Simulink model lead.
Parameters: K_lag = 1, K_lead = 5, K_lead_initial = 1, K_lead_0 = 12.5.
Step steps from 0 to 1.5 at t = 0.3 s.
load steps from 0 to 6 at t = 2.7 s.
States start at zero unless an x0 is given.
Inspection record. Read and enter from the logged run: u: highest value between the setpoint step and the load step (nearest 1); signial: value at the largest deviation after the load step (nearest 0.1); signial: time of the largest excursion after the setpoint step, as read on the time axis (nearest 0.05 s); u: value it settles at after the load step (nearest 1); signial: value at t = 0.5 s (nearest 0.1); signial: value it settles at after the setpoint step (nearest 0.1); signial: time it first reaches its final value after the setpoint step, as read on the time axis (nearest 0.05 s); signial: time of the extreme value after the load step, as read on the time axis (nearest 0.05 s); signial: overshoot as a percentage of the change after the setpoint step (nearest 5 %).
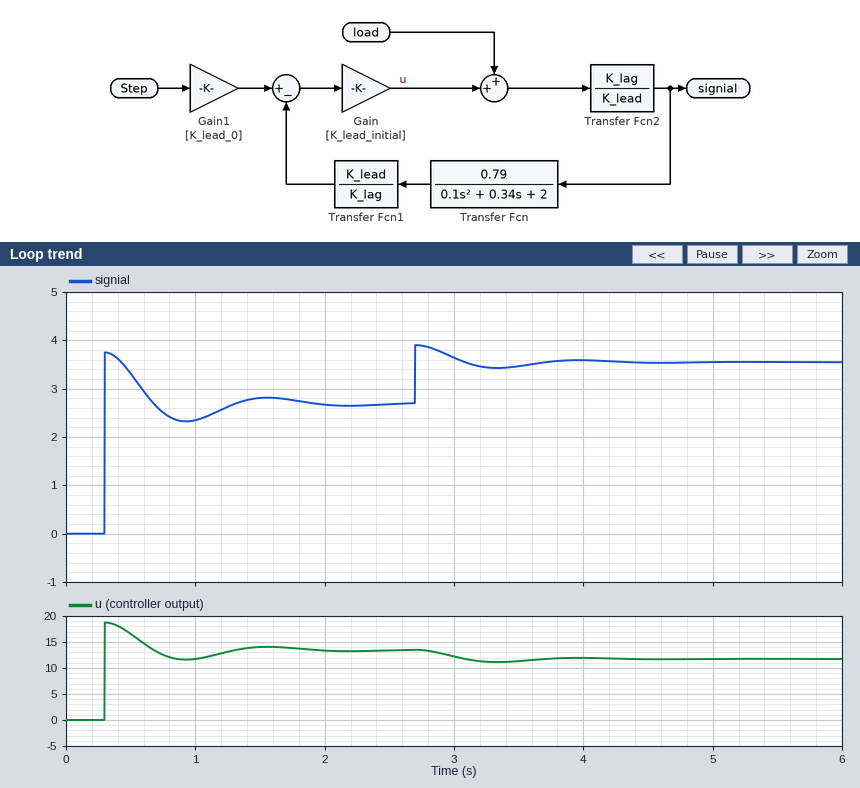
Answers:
19
3.9
0.30 s
12
3.3
2.7
0.30 s
2.70 s
40 %
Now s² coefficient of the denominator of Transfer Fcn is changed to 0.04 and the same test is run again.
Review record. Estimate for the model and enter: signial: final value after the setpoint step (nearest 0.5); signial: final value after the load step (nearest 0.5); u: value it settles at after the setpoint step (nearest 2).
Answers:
2.5
3.5
14
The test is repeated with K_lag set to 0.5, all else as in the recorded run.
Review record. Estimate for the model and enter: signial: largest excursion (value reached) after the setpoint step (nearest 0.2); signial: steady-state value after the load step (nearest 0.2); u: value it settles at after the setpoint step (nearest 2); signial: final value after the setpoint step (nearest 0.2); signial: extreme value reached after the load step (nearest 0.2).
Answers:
1.8
1.8
14
1.4
2.0
